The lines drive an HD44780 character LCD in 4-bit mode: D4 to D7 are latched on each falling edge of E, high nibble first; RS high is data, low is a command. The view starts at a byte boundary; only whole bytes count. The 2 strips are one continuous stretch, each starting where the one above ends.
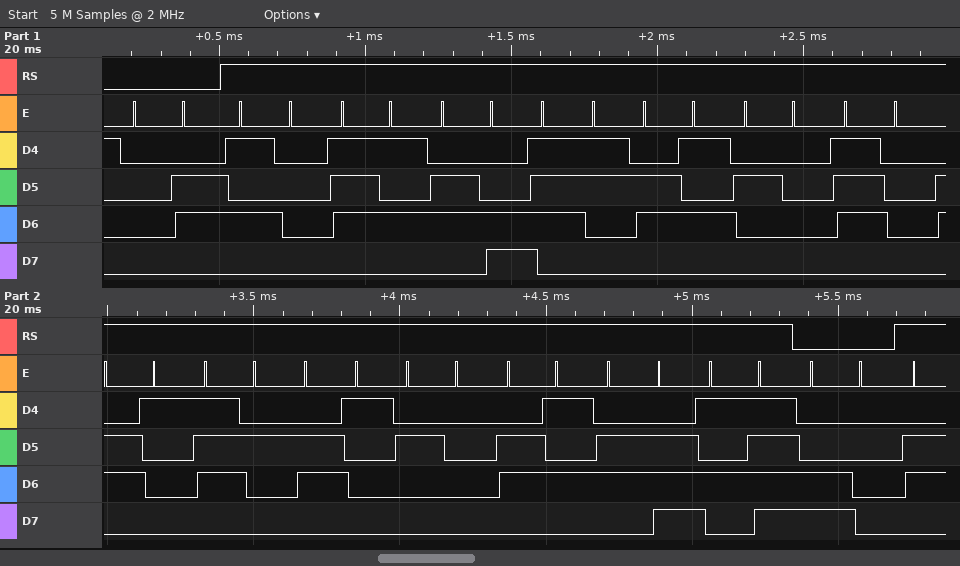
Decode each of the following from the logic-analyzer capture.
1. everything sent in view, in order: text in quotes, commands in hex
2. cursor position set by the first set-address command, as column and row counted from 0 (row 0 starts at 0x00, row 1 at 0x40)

0x06 "Pulse para en_" 0xC0
column 0, row 1
